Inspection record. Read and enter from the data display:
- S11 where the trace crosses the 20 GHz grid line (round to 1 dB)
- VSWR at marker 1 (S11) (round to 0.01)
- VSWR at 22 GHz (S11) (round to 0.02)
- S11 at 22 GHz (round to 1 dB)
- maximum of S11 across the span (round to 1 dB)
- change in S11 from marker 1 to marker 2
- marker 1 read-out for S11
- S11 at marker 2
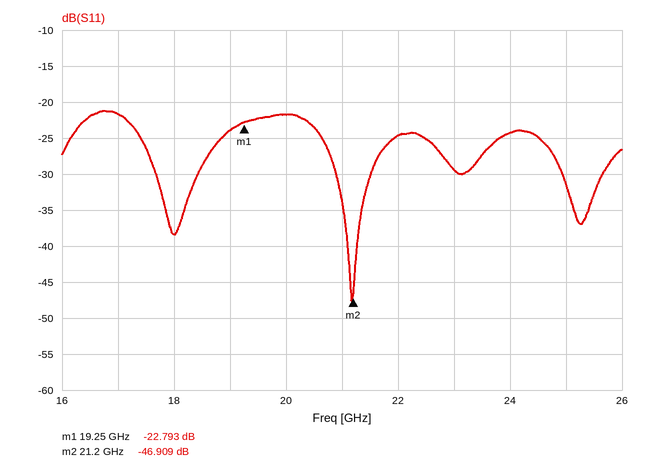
-22 dB
1.16
1.12
-25 dB
-21 dB
-24.116 dB
-22.793 dB
-46.909 dB
